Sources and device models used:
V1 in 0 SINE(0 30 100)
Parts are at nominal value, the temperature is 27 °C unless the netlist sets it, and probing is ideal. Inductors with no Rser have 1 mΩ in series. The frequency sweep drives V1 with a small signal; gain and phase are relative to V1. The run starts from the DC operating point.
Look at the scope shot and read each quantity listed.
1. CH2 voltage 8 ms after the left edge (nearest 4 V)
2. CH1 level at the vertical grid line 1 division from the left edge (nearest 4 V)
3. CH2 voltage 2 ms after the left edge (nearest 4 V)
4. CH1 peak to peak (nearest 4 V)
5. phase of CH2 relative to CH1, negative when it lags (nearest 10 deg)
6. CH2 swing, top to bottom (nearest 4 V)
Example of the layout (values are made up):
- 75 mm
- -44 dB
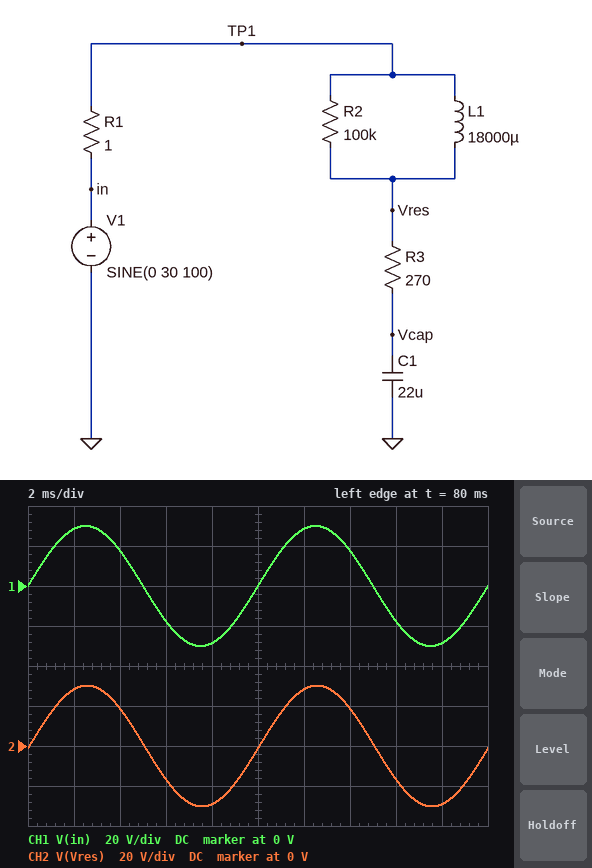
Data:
- -28 V
- 28 V
- 28 V
- 60 V
- 0 deg
- 60 V
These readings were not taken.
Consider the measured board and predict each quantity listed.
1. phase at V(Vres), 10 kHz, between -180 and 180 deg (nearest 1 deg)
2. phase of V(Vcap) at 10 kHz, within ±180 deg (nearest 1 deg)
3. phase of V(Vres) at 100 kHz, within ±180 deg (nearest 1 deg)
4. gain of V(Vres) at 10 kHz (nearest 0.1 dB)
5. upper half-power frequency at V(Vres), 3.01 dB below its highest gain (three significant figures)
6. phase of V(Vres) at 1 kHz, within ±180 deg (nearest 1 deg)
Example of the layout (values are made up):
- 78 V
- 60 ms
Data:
- -76 deg
- -166 deg
- -82 deg
- -12.7 dB
- 2.37 kHz
- -23 deg
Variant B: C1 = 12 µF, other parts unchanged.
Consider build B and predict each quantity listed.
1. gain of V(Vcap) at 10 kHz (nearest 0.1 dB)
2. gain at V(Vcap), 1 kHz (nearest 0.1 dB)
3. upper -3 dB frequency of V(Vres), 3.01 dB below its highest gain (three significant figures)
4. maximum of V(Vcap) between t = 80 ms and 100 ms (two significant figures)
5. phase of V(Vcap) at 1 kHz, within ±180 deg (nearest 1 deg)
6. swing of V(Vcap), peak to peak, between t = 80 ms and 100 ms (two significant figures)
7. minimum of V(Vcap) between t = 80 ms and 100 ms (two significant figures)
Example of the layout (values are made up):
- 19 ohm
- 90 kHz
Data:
- -58.9 dB
- -26.8 dB
- 2.36 kHz
- 13 V
- -110 deg
- 27 V
- -13 V
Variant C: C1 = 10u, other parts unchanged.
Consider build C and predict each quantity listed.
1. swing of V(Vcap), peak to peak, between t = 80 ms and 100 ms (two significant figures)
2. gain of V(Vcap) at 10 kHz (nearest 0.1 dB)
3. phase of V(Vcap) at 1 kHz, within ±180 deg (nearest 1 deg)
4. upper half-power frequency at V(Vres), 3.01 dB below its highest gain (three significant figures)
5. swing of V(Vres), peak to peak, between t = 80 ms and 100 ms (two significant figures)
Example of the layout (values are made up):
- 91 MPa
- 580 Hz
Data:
- 31 V
- -57.3 dB
- -110 deg
- 2.35 kHz
- 61 V
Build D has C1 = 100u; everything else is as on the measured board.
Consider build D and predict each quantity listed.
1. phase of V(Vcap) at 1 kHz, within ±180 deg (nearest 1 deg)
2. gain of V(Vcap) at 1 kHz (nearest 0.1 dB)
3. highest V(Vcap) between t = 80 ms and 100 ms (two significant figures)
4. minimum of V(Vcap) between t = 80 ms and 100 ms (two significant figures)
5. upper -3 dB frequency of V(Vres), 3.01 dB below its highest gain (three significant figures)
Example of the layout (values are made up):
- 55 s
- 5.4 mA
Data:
- -112 deg
- -45.3 dB
- 1.8 V
- -1.7 V
- 2.38 kHz
